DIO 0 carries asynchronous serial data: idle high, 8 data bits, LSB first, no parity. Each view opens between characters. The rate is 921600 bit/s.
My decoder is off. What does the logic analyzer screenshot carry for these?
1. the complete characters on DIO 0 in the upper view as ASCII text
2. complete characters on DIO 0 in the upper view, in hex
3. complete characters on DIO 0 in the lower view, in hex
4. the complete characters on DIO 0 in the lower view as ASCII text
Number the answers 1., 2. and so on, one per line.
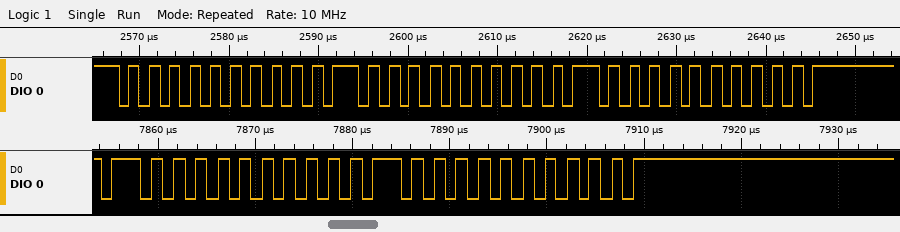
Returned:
1. "UUWUuUU"
2. 55, 55, 57, 55, 75, 55, 55
3. 57, 55, 75, 55, 55
4. "WUuUU"
